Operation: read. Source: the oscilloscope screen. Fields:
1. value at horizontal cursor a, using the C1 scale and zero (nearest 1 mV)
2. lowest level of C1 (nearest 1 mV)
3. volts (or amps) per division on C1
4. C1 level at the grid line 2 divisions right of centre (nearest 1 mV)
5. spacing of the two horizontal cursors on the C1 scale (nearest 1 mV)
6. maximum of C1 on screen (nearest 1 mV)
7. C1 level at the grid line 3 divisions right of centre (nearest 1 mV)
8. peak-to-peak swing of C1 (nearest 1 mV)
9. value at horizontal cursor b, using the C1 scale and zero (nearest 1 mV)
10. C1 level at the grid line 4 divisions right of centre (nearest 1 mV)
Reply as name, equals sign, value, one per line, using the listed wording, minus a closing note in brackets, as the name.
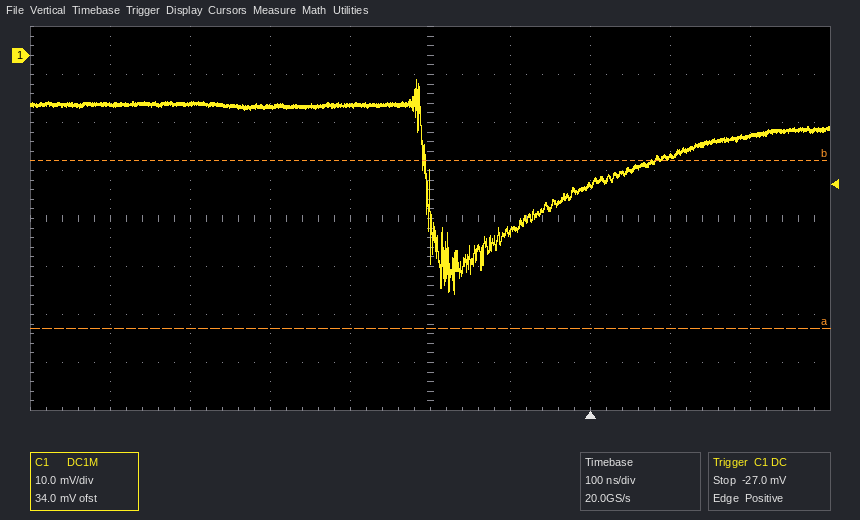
value at horizontal cursor a, using the C1 scale and zero = -57 mV
lowest level of C1 = -50 mV
volts (or amps) per division on C1 = 10 mV
C1 level at the grid line 2 divisions right of centre = -27 mV
spacing of the two horizontal cursors on the C1 scale = 35 mV
maximum of C1 on screen = -5 mV
C1 level at the grid line 3 divisions right of centre = -21 mV
peak-to-peak swing of C1 = 45 mV
value at horizontal cursor b, using the C1 scale and zero = -22 mV
C1 level at the grid line 4 divisions right of centre = -17 mV
